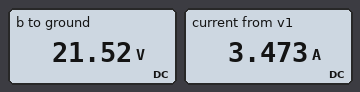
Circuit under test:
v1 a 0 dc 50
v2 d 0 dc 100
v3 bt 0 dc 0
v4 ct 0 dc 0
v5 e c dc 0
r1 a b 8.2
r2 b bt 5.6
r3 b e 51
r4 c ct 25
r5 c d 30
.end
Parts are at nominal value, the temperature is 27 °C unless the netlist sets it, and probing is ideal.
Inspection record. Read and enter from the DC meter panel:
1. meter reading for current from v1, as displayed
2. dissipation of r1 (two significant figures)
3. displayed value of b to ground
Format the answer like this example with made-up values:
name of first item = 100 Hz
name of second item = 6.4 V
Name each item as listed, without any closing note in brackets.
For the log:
meter reading for current from v1, as displayed = 3.473 A
dissipation of r1 = 99 W
displayed value of b to ground = 21.52 V
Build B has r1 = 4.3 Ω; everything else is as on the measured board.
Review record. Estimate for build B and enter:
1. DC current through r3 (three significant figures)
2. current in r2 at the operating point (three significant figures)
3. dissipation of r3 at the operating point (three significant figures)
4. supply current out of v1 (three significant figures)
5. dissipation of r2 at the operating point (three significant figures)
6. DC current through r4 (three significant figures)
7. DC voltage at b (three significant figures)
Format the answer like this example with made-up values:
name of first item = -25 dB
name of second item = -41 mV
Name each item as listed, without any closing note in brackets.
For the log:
DC current through r3 = 256 mA
current in r2 at the operating point = 5.16 A
dissipation of r3 at the operating point = 3.34 W
supply current out of v1 = 4.91 A
dissipation of r2 at the operating point = 149 W
DC current through r4 = 1.68 A
DC voltage at b = 28.9 V
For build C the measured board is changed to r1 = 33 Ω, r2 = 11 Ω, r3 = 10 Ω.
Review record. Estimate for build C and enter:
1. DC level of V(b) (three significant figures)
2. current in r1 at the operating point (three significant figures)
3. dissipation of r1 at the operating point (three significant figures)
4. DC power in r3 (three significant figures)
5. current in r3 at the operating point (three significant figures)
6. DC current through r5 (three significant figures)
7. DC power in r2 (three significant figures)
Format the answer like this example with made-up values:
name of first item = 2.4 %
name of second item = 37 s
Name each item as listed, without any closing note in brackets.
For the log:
DC level of V(b) = 21.0 V
current in r1 at the operating point = 878 mA
dissipation of r1 at the operating point = 25.4 W
DC power in r3 = 10.7 W
current in r3 at the operating point = 1.03 A
DC current through r5 = 2.29 A
DC power in r2 = 40.2 W
